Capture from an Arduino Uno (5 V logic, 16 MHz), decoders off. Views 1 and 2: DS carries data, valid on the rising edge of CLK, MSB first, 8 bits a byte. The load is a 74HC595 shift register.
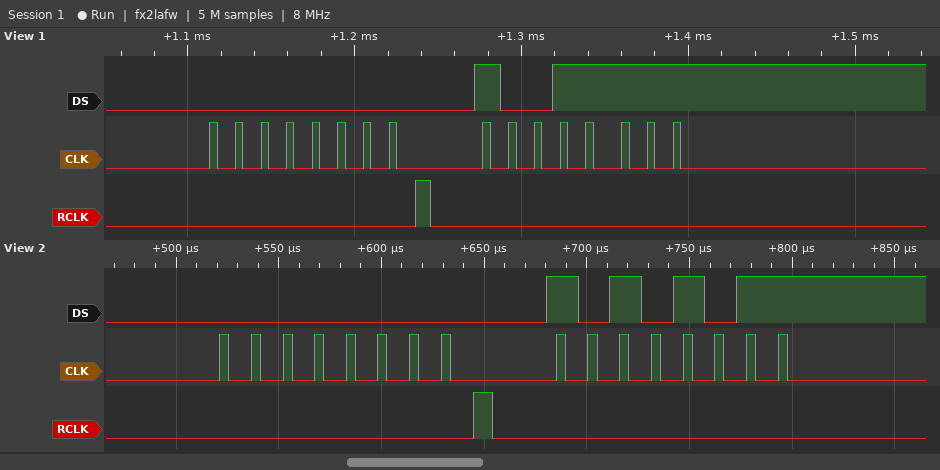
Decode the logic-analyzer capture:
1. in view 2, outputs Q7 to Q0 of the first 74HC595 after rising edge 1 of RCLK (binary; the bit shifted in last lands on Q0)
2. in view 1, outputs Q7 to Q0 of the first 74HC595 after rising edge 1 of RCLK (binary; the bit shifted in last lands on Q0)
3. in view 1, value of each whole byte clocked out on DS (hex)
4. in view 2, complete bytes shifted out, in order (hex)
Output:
00000000
00000000
00 9F
00 AB
